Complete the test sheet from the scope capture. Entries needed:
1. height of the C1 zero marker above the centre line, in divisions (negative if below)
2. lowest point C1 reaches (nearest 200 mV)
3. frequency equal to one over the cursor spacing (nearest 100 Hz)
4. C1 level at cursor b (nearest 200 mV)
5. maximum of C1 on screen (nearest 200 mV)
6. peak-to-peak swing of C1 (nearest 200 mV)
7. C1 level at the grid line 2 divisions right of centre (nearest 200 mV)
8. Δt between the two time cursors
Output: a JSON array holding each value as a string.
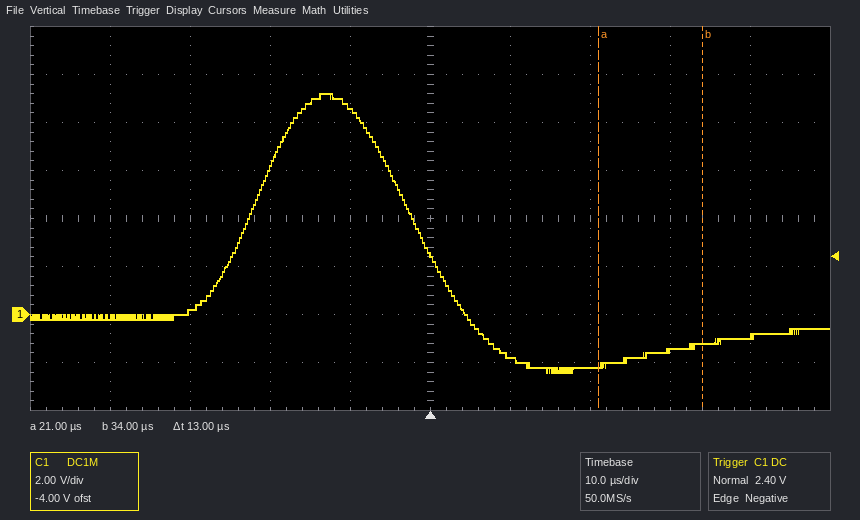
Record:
["-2.0 div", "-2.4 V", "76.9 kHz", "-1.2 V", "9.2 V", "11.6 V", "-2.2 V", "13 µs"]
